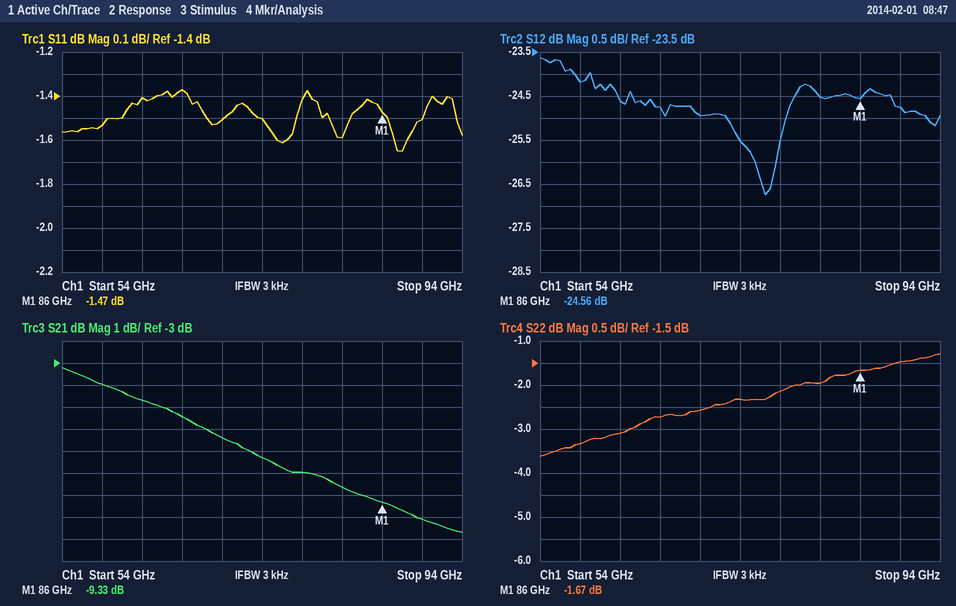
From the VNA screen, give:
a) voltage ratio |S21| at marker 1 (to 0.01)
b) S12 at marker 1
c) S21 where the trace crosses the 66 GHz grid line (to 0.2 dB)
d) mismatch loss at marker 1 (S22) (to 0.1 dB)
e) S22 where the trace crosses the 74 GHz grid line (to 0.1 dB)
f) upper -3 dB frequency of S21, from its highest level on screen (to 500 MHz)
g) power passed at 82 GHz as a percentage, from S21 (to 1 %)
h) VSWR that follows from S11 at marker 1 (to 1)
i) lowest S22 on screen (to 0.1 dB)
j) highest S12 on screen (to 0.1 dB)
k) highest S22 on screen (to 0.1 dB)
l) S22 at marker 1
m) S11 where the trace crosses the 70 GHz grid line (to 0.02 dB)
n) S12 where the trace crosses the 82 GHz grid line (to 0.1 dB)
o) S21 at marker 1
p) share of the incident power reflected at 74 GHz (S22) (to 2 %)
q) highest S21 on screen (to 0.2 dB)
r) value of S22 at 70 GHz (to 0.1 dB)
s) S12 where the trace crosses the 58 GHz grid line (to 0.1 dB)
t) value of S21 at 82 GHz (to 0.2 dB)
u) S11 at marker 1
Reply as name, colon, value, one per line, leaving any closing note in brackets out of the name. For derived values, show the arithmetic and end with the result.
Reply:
voltage ratio |S21| at marker 1: 10^(-9.33/20) ≈ 0.34
S12 at marker 1: -24.56 dB
S21 where the trace crosses the 66 GHz grid line: -5.4 dB
mismatch loss at marker 1 (S22): −10 log10(1 − 10^(-1.67/10)) ≈ 5.0 dB
S22 where the trace crosses the 74 GHz grid line: -2.3 dB
upper -3 dB frequency of S21, from its highest level on screen: 69.0 GHz
power passed at 82 GHz as a percentage, from S21: 10^(-8.6/10) ≈ 14 %
VSWR that follows from S11 at marker 1: (1 + 0.8443)/(1 − 0.8443) ≈ 12
lowest S22 on screen: -3.6 dB
highest S12 on screen: -23.6 dB
highest S22 on screen: -1.3 dB
S22 at marker 1: -1.67 dB
S11 where the trace crosses the 70 GHz grid line: -1.50 dB
S12 where the trace crosses the 82 GHz grid line: -24.5 dB
S21 at marker 1: -9.33 dB
share of the incident power reflected at 74 GHz (S22): 10^(-2.3/10) ≈ 58.9 %, so 58 % to the nearest 2 %
highest S21 on screen: -3.2 dB
value of S22 at 70 GHz: -2.6 dB
S12 where the trace crosses the 58 GHz grid line: -24.2 dB
value of S21 at 82 GHz: -8.6 dB
S11 at marker 1: -1.47 dB
